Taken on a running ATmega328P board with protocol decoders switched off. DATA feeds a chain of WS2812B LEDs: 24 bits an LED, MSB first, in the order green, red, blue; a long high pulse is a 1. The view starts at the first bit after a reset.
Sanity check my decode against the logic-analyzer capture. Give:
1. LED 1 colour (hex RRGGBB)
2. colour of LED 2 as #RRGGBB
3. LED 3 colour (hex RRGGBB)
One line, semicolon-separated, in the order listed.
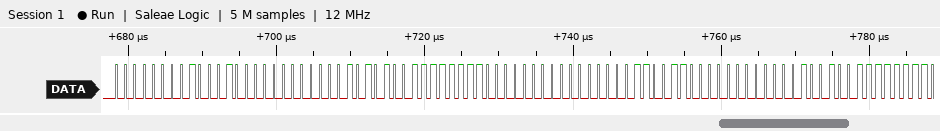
#880000; #FF5400; #CC0000
